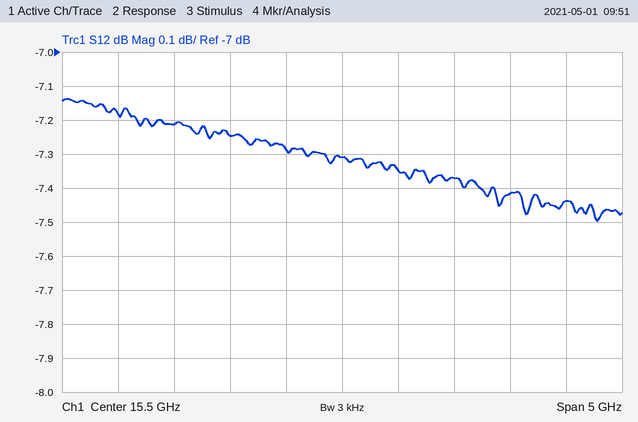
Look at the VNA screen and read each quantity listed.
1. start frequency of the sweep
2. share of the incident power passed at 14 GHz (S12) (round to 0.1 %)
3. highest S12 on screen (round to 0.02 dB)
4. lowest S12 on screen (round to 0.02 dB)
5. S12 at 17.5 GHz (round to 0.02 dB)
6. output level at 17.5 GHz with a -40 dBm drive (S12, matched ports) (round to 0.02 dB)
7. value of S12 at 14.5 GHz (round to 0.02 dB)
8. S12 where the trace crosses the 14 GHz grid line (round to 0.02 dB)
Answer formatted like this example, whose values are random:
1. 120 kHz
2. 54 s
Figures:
1. 13 GHz
2. 19.0 %
3. -7.14 dB
4. -7.50 dB
5. -7.44 dB
6. -47.44 dBm
7. -7.24 dB
8. -7.22 dB
